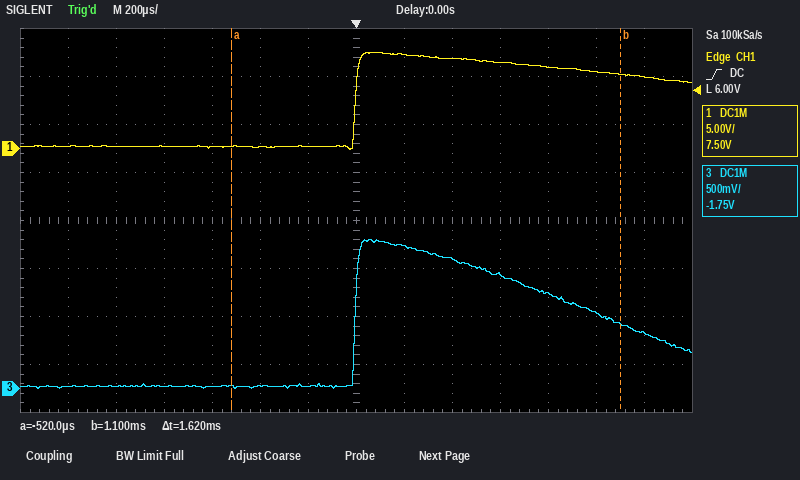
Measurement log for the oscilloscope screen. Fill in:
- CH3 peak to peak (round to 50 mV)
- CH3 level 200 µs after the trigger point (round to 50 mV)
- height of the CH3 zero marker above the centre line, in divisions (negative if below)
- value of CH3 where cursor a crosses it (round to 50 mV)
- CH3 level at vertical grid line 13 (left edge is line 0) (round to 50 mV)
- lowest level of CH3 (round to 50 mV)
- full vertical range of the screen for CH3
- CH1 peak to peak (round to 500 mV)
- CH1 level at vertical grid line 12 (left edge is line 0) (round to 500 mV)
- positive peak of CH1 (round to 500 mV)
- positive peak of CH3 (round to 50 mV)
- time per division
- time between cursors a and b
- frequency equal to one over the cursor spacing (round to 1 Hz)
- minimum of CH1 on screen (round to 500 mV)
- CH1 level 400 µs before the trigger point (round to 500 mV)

1.55 V
1.50 V
-3.5 div
0 mV
600 mV
0 mV
4 V
10.0 V
8.0 V
10.0 V
1.55 V
200 µs
1.62 ms
617 Hz
0.0 V
0.0 V
